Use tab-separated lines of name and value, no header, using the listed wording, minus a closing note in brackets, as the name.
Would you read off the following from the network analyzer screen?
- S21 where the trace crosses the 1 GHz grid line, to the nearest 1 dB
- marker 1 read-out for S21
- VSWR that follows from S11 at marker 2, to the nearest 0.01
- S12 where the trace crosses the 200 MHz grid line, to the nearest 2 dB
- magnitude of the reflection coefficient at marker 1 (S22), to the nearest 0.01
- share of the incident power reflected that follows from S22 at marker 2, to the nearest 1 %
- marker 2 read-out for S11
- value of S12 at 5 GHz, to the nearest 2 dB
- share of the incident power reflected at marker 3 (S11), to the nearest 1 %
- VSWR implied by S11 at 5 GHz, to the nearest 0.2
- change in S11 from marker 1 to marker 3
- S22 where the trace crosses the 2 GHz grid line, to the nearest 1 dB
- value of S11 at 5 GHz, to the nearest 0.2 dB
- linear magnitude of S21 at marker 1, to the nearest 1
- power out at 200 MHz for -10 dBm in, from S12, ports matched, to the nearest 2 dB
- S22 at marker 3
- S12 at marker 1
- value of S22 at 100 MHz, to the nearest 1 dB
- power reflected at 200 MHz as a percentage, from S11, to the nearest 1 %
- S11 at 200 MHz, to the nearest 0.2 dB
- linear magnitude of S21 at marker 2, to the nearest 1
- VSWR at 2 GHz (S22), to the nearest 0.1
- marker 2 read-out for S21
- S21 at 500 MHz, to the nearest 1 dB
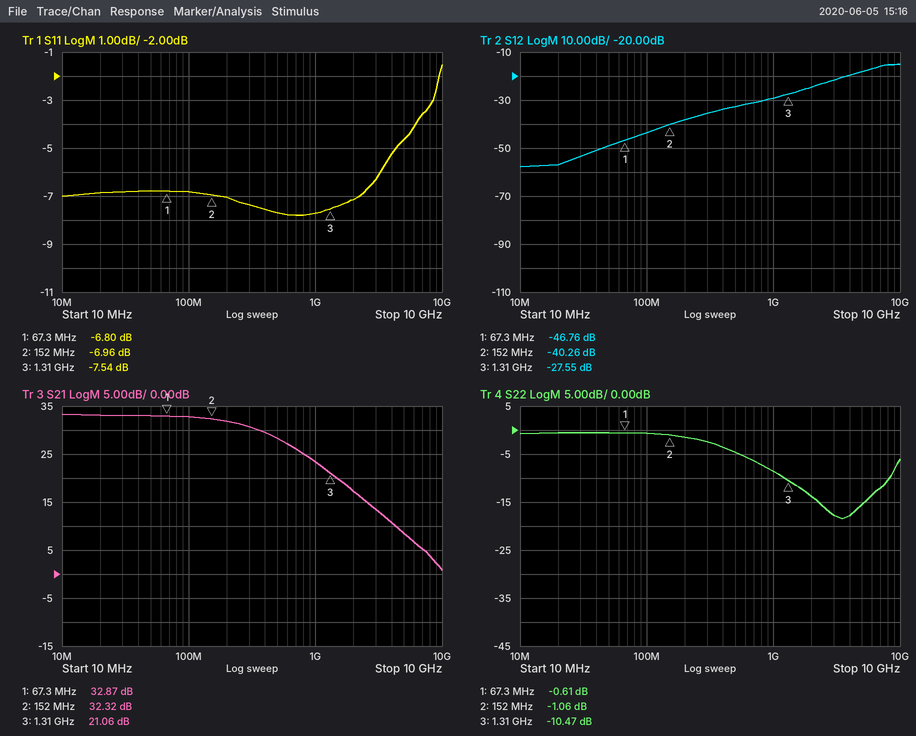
S21 where the trace crosses the 1 GHz grid line, to the nearest 1 dB	23 dB
marker 1 read-out for S21	32.87 dB
VSWR that follows from S11 at marker 2, to the nearest 0.01	2.63
S12 where the trace crosses the 200 MHz grid line, to the nearest 2 dB	-38 dB
magnitude of the reflection coefficient at marker 1 (S22), to the nearest 0.01	0.93
share of the incident power reflected that follows from S22 at marker 2, to the nearest 1 %	78 %
marker 2 read-out for S11	-6.96 dB
value of S12 at 5 GHz, to the nearest 2 dB	-18 dB
share of the incident power reflected at marker 3 (S11), to the nearest 1 %	18 %
VSWR implied by S11 at 5 GHz, to the nearest 0.2	3.8
change in S11 from marker 1 to marker 3	-0.74 dB
S22 where the trace crosses the 2 GHz grid line, to the nearest 1 dB	-14 dB
value of S11 at 5 GHz, to the nearest 0.2 dB	-4.6 dB
linear magnitude of S21 at marker 1, to the nearest 1	44
power out at 200 MHz for -10 dBm in, from S12, ports matched, to the nearest 2 dB	-48 dBm
S22 at marker 3	-10.47 dB
S12 at marker 1	-46.76 dB
value of S22 at 100 MHz, to the nearest 1 dB	-1 dB
power reflected at 200 MHz as a percentage, from S11, to the nearest 1 %	20 %
S11 at 200 MHz, to the nearest 0.2 dB	-7.0 dB
linear magnitude of S21 at marker 2, to the nearest 1	41
VSWR at 2 GHz (S22), to the nearest 0.1	1.5
marker 2 read-out for S21	32.32 dB
S21 at 500 MHz, to the nearest 1 dB	28 dB
